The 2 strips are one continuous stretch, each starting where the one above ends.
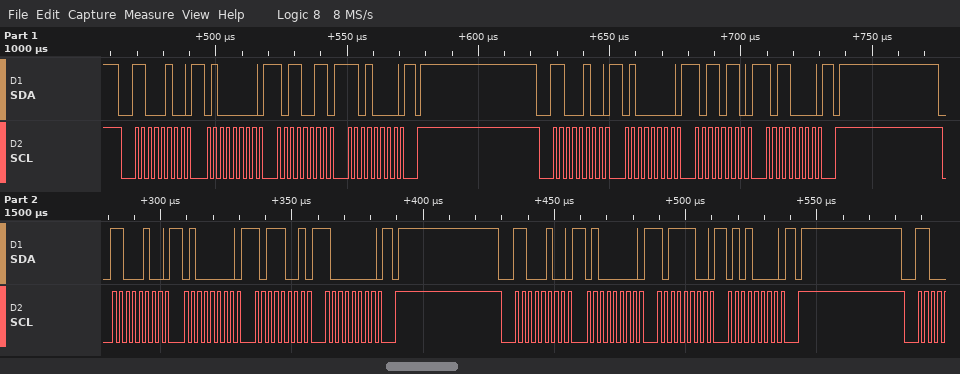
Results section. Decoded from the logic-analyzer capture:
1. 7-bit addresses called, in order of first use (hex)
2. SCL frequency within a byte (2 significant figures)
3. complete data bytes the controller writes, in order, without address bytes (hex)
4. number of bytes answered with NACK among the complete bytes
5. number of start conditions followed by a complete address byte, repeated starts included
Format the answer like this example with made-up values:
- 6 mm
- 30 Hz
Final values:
- 0x62
- 400 kHz
- 40 B3 D0 40 B6 B0 40 B9 80 40 BC 50
- 0
- 4
